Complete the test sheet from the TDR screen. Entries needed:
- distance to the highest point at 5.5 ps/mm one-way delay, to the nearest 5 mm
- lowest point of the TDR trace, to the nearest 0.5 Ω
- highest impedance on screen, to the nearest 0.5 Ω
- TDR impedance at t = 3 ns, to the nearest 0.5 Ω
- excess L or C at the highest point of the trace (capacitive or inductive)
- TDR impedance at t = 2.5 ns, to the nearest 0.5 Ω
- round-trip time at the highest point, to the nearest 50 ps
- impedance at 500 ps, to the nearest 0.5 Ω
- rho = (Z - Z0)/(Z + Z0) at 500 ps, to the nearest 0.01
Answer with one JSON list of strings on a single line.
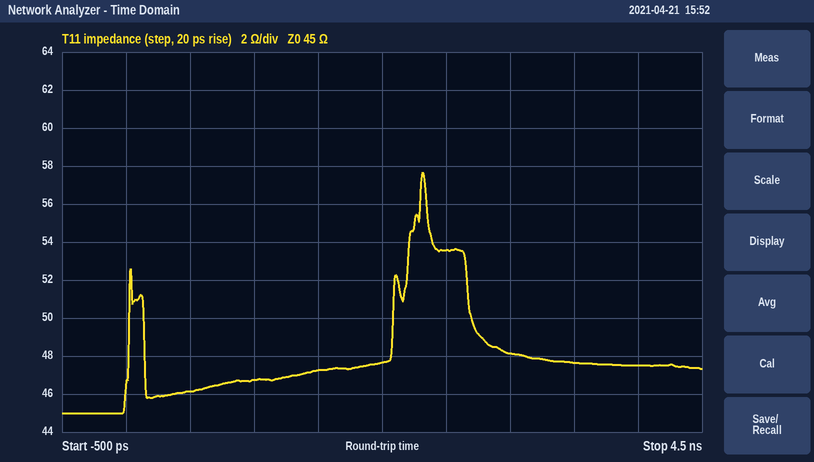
["210 mm", "45.0 Ω", "57.5 Ω", "48.0 Ω", "inductive", "53.5 Ω", "2.30 ns", "46.0 Ω", "+0.01"]
